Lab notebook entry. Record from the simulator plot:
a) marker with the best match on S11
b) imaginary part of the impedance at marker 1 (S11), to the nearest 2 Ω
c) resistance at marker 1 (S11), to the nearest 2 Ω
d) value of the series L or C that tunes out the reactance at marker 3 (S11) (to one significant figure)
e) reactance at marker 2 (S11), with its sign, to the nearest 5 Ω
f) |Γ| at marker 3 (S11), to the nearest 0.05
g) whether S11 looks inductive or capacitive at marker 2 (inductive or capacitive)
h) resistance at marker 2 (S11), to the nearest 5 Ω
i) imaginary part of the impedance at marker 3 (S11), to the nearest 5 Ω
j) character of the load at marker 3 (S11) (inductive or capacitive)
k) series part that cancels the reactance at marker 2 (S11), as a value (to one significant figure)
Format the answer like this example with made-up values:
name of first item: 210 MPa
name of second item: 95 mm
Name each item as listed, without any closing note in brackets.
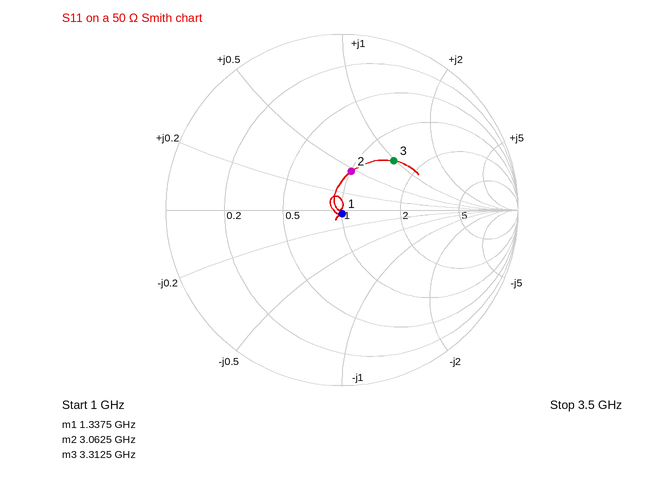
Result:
marker with the best match on S11: marker 1
imaginary part of the impedance at marker 1 (S11), to the nearest 2 Ω: -2 Ω
resistance at marker 1 (S11), to the nearest 2 Ω: 50 Ω
value of the series L or C that tunes out the reactance at marker 3 (S11): 1.0 pF
reactance at marker 2 (S11), with its sign, to the nearest 5 Ω: +25 Ω
|Γ| at marker 3 (S11), to the nearest 0.05: 0.40
whether S11 looks inductive or capacitive at marker 2: inductive
resistance at marker 2 (S11), to the nearest 5 Ω: 50 Ω
imaginary part of the impedance at marker 3 (S11), to the nearest 5 Ω: +50 Ω
character of the load at marker 3 (S11): inductive
series part that cancels the reactance at marker 2 (S11), as a value: 2 pF
